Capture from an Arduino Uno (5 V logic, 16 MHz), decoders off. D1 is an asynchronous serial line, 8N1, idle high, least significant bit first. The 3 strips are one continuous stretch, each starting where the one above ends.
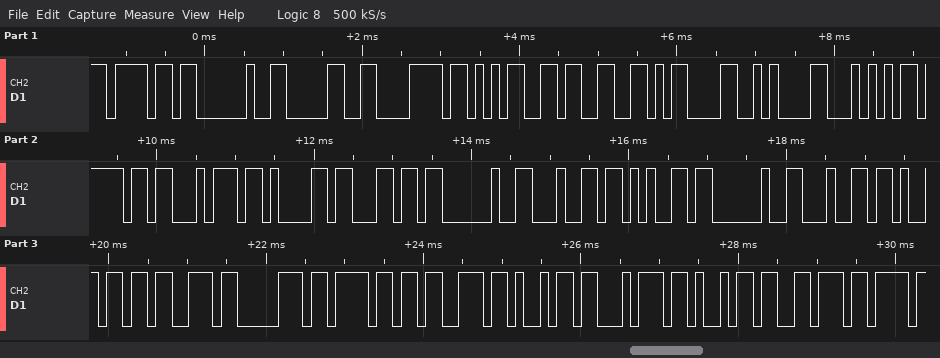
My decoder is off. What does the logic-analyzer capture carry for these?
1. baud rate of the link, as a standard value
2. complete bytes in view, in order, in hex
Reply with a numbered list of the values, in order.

1. 9600 baud
2. 0x6F 0x20 0x30 0x78 0x35 0x33 0x0D 0x0A 0x54 0x6F 0x74 0x61 0x6C 0x20 0x64 0x65 0x20 0x64 0x69 0x73 0x70 0x6F 0x73 0x69 0x74 0x69 0x76
